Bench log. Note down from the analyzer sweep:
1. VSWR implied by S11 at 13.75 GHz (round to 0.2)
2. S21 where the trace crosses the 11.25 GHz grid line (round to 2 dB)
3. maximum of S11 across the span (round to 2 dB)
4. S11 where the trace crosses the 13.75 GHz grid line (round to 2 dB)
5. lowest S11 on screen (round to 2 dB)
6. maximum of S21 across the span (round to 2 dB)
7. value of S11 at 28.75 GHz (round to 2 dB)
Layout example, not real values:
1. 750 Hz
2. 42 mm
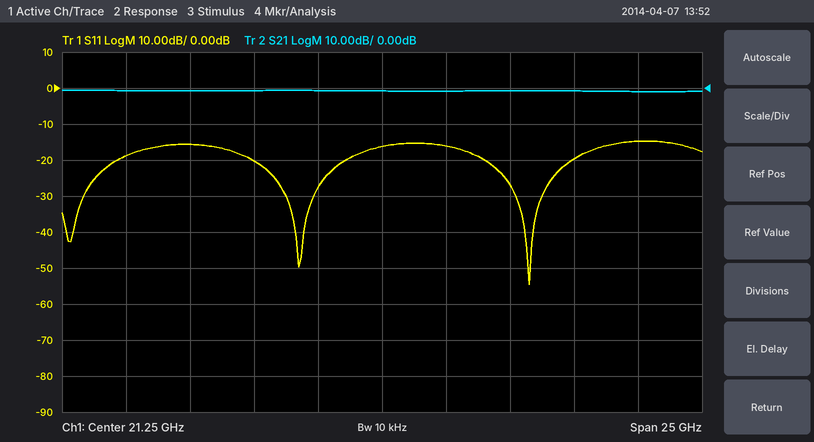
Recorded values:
1. 1.4
2. 0 dB
3. -14 dB
4. -16 dB
5. -54 dB
6. 0 dB
7. -20 dB
